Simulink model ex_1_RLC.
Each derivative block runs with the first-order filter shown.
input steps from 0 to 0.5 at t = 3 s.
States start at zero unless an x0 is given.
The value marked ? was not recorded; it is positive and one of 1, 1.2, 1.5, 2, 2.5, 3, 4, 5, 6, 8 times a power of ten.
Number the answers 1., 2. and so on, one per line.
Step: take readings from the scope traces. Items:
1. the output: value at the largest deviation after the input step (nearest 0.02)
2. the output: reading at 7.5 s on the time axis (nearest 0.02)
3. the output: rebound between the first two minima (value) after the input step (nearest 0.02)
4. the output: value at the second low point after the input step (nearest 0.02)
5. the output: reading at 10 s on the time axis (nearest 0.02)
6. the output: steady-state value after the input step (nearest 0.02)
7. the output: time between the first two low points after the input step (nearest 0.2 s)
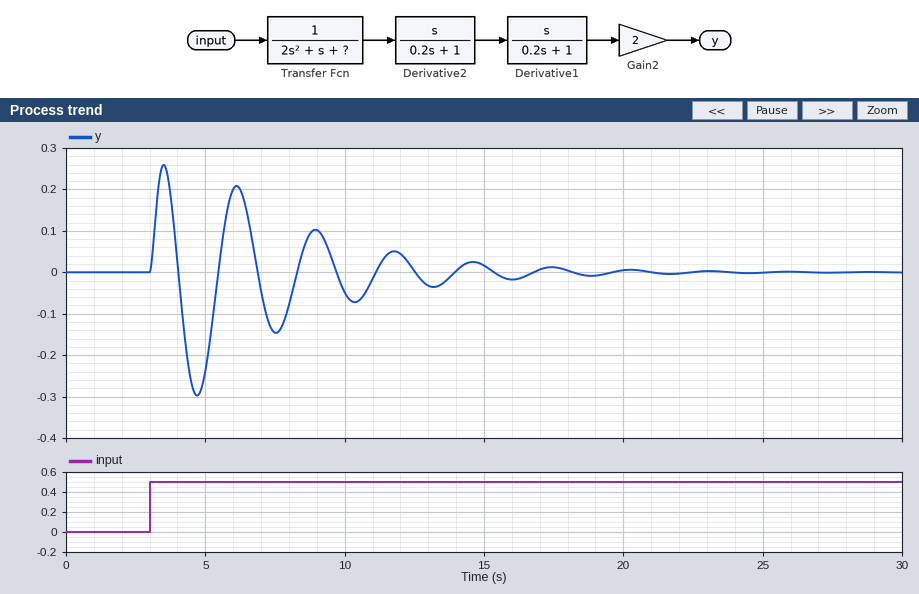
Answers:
1. -0.30
2. -0.14
3. 0.20
4. -0.14
5. -0.04
6. 0.00
7. 2.8 s
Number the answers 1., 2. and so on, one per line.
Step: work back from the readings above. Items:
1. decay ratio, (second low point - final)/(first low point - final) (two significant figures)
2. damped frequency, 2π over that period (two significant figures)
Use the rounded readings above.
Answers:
1. 0.47
2. 2.2 rad/s
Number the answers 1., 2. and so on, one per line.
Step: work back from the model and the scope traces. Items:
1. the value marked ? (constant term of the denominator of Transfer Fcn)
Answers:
1. 10
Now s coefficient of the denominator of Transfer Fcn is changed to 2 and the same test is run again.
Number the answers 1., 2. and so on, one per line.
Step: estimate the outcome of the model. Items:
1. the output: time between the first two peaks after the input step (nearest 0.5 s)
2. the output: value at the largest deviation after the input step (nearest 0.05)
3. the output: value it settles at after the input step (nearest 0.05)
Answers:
1. 2.5 s
2. 0.25
3. 0.00
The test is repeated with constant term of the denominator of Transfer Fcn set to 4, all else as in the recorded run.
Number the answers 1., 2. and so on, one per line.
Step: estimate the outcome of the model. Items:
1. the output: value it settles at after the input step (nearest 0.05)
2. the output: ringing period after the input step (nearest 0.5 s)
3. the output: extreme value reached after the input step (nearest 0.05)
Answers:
1. 0.00
2. 4.0 s
3. 0.30
